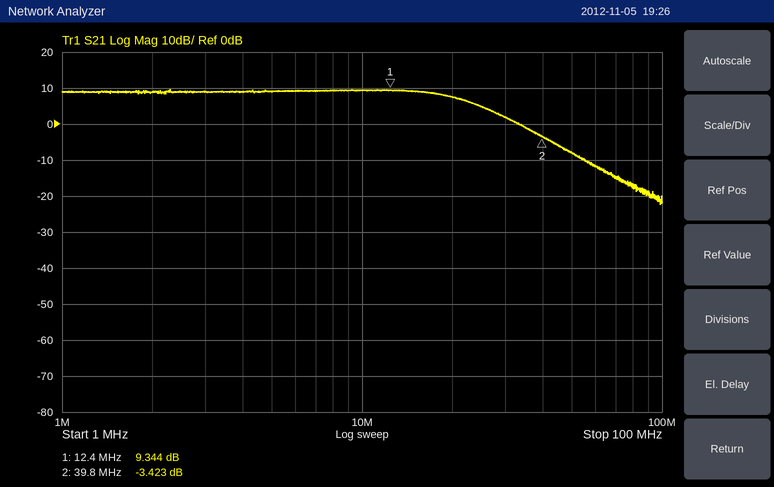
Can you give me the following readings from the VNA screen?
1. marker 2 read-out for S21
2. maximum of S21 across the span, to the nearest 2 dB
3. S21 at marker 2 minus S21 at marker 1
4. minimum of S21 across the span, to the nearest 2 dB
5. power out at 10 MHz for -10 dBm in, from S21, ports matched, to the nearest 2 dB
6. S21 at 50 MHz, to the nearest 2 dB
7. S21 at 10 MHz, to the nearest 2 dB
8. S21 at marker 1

-3.423 dB
10 dB
-12.767 dB
-22 dB
0 dBm
-8 dB
10 dB
9.344 dB
